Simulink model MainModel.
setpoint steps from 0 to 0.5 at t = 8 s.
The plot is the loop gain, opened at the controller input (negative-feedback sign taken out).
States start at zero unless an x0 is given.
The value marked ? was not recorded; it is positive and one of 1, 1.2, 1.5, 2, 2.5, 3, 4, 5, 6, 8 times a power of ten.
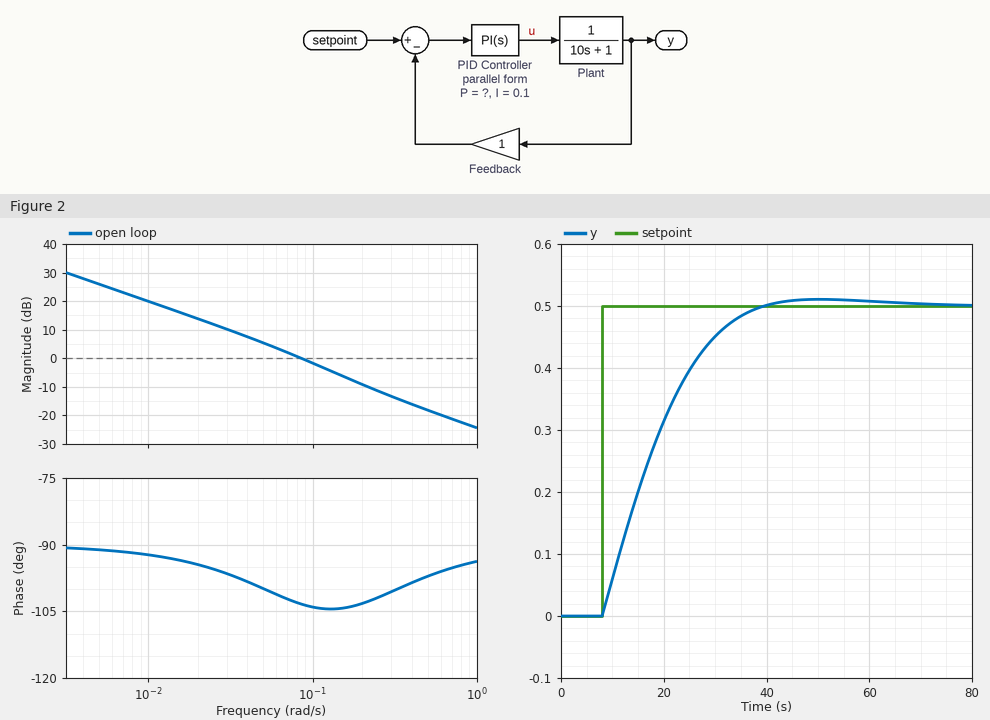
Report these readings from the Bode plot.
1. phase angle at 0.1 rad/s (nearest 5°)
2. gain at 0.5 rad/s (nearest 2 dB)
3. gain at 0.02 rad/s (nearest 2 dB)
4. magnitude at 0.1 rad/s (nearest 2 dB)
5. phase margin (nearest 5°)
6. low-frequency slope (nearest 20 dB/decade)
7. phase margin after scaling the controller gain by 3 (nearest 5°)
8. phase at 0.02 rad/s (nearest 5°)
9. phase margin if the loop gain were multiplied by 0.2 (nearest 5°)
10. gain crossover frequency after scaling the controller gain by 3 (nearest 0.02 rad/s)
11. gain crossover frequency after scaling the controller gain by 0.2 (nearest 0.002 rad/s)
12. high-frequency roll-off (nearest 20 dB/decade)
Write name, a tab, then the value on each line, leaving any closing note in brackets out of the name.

phase angle at 0.1 rad/s	-105°
gain at 0.5 rad/s	-18 dB
gain at 0.02 rad/s	14 dB
magnitude at 0.1 rad/s	-2 dB
phase margin	75°
low-frequency slope	-20 dB/decade
phase margin after scaling the controller gain by 3	75°
phase at 0.02 rad/s	-95°
phase margin if the loop gain were multiplied by 0.2	85°
gain crossover frequency after scaling the controller gain by 3	0.20 rad/s
gain crossover frequency after scaling the controller gain by 0.2	0.020 rad/s
high-frequency roll-off	-20 dB/decade
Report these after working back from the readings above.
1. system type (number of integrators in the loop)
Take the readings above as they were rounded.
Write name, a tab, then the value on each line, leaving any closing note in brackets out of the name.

system type	1
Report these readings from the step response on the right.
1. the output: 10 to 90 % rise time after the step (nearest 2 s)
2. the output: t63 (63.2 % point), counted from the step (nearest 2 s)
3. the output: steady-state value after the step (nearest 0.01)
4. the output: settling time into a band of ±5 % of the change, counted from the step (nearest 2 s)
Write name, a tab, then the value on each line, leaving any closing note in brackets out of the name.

the output: 10 to 90 % rise time after the step	20 s
the output: t63 (63.2 % point), counted from the step	12 s
the output: steady-state value after the step	0.50
the output: settling time into a band of ±5 % of the change, counted from the step	26 s
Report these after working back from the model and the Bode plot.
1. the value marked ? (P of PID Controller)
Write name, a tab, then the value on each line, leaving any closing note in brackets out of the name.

the value marked ?	0.6
